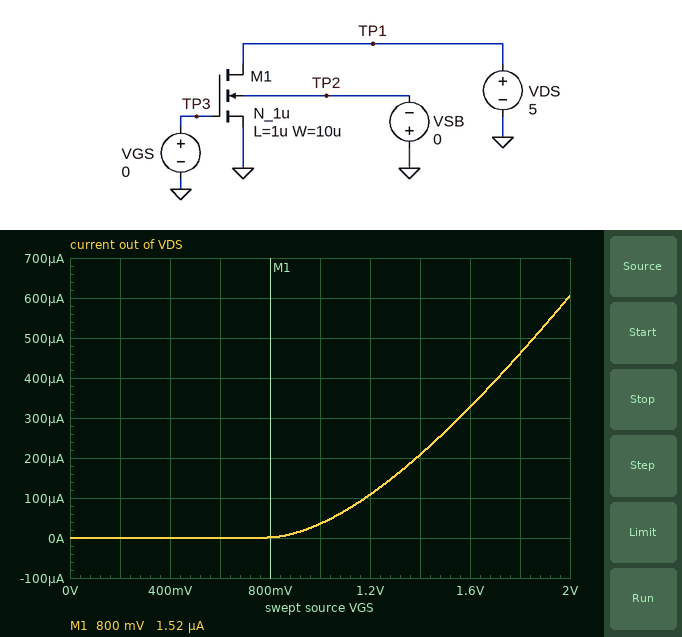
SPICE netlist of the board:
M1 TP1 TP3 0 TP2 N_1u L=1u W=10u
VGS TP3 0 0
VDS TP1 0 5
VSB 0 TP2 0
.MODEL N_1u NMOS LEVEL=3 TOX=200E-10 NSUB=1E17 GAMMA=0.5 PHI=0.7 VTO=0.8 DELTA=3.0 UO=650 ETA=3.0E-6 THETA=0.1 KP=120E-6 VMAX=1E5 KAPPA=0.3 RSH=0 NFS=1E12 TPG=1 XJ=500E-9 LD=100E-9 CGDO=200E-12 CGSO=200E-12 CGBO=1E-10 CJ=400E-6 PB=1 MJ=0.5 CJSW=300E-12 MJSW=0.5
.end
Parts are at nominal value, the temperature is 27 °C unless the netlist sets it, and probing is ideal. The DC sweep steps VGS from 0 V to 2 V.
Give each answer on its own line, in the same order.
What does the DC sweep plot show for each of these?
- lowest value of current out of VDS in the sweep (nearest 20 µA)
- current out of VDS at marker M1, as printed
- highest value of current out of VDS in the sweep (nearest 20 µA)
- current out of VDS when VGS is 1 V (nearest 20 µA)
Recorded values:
0 A
1.52 µA
600 µA
40 µA
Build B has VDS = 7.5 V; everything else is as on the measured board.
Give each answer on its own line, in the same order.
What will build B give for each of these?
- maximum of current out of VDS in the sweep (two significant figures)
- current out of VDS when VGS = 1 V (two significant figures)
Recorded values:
640 µA
37 µA
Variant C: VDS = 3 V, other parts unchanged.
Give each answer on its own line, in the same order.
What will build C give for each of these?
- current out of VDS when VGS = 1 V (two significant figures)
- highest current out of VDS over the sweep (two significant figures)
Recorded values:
34 µA
580 µA
